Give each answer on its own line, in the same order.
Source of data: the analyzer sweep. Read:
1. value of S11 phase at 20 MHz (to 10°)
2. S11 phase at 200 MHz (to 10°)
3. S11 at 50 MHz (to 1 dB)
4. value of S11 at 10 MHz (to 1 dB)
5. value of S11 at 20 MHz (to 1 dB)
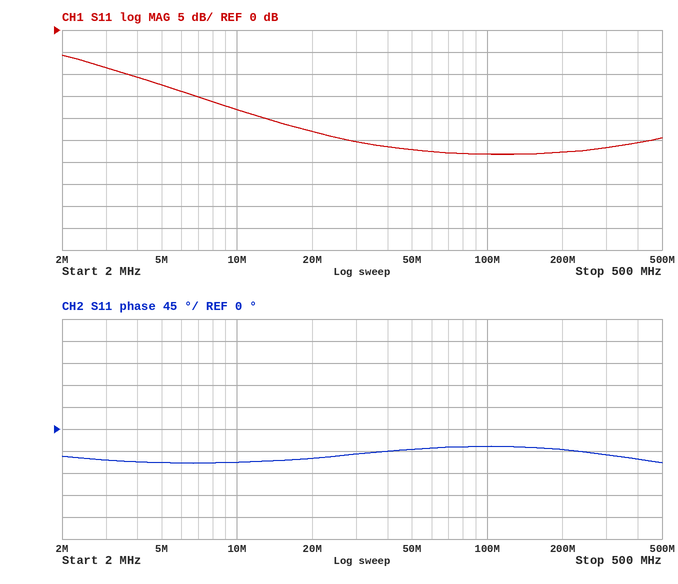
-60°
-40°
-27 dB
-18 dB
-23 dB
